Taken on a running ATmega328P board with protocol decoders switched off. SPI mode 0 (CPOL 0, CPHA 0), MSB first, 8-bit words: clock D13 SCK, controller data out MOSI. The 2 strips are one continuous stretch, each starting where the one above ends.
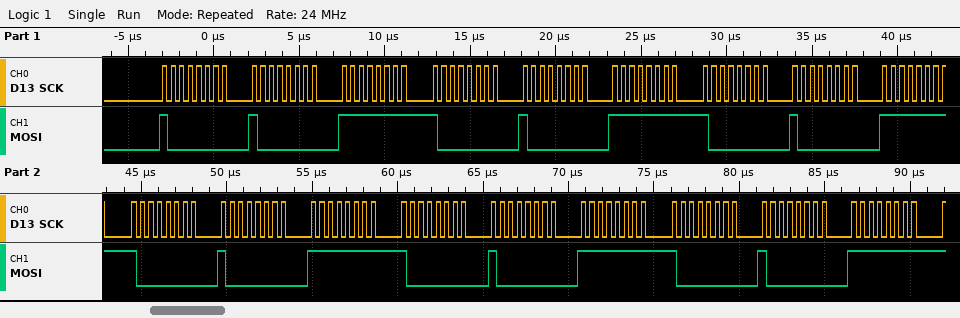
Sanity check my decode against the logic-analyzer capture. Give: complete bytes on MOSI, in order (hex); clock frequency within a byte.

80 80 FF 80 80 FF 80 80 FF 80 80 FF 80 80 FF 80 80 FF
2 MHz
